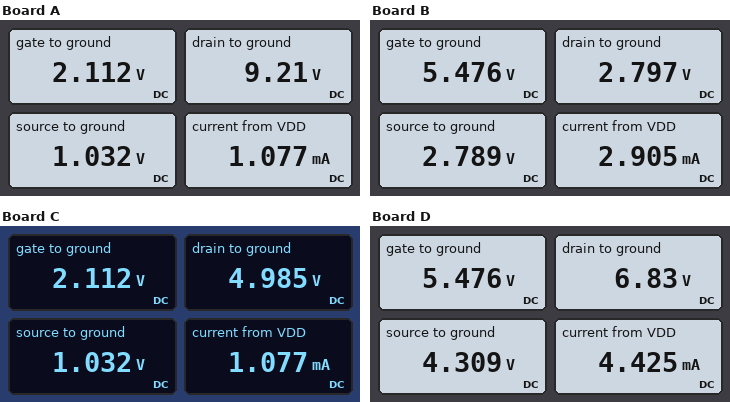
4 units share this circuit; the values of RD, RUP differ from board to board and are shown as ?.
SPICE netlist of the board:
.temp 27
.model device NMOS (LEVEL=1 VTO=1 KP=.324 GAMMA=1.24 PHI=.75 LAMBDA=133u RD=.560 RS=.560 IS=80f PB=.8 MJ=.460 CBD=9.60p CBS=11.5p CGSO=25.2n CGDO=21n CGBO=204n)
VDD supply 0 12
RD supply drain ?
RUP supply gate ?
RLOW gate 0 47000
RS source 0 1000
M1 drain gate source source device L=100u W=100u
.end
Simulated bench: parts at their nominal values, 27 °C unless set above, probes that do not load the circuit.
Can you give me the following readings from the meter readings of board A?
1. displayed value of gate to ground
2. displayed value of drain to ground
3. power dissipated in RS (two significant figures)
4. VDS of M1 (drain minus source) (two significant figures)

2.112 V
9.21 V
1.1 mW
8.2 V
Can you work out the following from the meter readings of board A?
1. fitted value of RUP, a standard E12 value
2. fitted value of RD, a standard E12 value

220 kΩ
2.7 kΩ
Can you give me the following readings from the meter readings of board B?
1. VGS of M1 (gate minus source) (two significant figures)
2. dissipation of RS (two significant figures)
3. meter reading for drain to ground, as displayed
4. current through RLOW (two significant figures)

2.7 V
7.8 mW
2.797 V
120 µA
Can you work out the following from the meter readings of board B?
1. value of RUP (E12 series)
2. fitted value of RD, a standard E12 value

56 kΩ
3.3 kΩ
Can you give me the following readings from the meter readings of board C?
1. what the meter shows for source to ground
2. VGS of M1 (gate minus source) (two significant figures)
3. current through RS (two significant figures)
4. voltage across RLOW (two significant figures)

1.032 V
1.1 V
1.0 mA
2.1 V
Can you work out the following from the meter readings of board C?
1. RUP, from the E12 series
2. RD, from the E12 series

220 kΩ
6.8 kΩ
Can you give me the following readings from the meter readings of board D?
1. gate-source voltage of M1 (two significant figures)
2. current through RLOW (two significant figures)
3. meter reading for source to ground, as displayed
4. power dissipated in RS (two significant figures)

1.2 V
120 µA
4.309 V
19 mW
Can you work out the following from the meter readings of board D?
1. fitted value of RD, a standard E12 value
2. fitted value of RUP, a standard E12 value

1.2 kΩ
56 kΩ
